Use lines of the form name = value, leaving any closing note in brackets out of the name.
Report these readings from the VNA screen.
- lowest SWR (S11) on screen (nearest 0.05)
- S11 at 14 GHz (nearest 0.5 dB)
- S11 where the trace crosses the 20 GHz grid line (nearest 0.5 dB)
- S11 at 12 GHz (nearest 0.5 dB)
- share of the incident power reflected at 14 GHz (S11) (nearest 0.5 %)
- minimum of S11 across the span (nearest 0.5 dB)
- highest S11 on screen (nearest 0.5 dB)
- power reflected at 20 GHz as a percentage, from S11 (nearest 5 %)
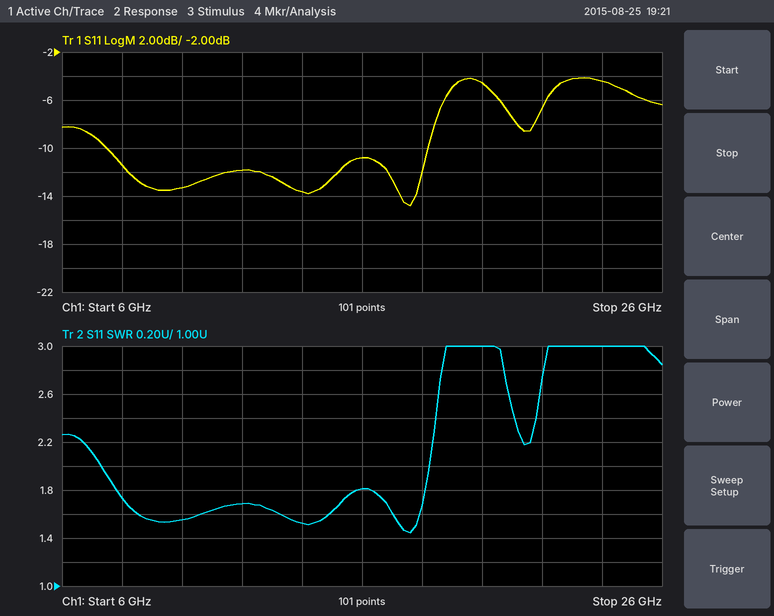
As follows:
lowest SWR (S11) on screen = 1.45
S11 at 14 GHz = -13.5 dB
S11 where the trace crosses the 20 GHz grid line = -4.5 dB
S11 at 12 GHz = -12.0 dB
share of the incident power reflected at 14 GHz (S11) = 4.5 %
minimum of S11 across the span = -15.0 dB
highest S11 on screen = -4.0 dB
power reflected at 20 GHz as a percentage, from S11 = 35 %
